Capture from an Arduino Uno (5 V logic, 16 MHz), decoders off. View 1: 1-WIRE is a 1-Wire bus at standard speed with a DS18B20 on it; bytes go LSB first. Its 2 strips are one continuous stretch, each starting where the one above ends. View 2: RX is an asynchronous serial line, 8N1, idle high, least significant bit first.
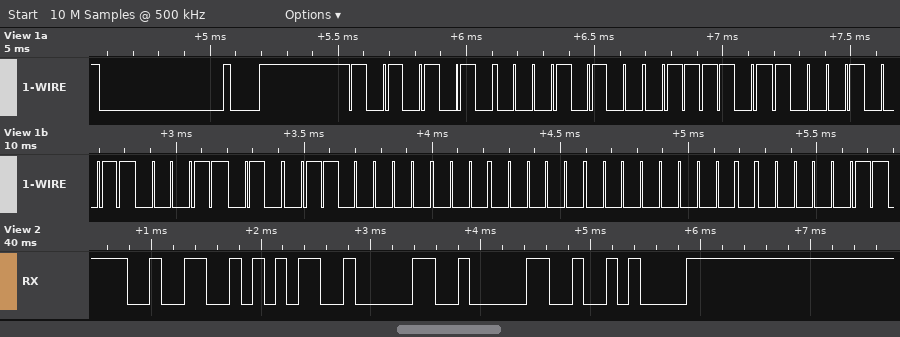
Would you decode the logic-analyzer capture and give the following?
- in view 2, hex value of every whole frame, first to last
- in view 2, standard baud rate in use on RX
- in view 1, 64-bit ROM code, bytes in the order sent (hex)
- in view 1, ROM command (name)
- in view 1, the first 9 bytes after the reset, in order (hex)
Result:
32 35 30 30 0A
9600 baud
28 DE C8 58 06 00 00 C0
Match ROM
55 28 DE C8 58 06 00 00 C0
